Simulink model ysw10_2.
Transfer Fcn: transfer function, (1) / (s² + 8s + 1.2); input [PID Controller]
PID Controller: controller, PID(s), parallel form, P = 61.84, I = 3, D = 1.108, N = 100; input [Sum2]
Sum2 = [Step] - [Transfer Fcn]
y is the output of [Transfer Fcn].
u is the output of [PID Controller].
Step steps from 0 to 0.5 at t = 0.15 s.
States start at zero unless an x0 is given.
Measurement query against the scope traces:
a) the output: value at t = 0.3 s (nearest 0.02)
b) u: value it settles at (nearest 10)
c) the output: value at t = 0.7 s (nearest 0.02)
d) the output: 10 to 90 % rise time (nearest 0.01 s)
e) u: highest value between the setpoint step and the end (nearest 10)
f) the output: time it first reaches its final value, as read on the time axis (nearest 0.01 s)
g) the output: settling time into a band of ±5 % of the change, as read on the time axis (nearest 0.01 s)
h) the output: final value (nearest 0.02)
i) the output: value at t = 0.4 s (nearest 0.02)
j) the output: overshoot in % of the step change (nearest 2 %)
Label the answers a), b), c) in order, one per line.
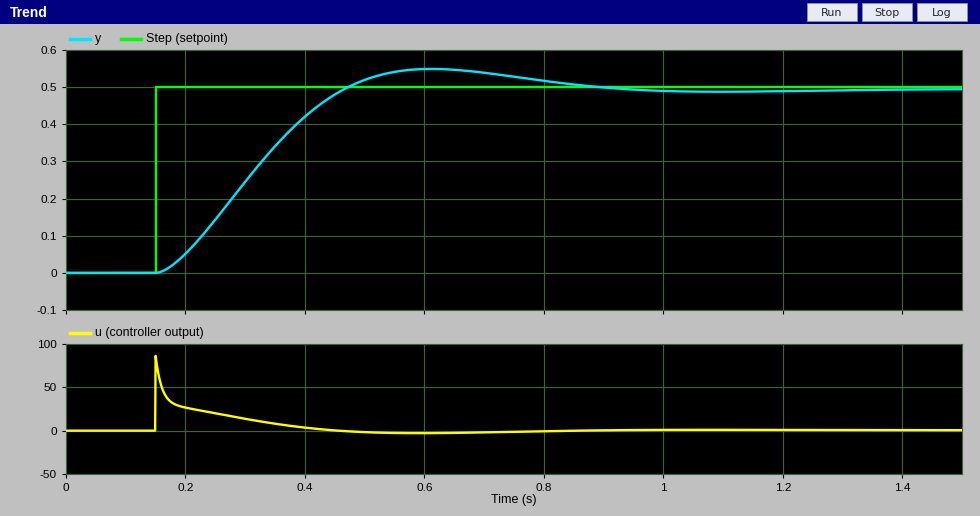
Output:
a) 0.24
b) 0
c) 0.54
d) 0.22 s
e) 90
f) 0.47 s
g) 0.79 s
h) 0.50
i) 0.42
j) 10 %
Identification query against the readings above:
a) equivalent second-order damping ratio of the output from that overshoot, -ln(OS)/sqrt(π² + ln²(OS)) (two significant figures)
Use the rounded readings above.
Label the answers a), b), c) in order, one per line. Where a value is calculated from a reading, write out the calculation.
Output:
a) ln(0.1) = -2.303; 2.303 / sqrt(9.870 + 5.302) = 0.59
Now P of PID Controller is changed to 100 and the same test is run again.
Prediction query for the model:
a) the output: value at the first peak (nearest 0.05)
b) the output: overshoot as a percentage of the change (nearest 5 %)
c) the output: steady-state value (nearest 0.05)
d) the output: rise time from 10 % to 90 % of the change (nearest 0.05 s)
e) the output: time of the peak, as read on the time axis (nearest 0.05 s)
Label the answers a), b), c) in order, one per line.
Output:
a) 0.60
b) 20 %
c) 0.50
d) 0.15 s
e) 0.50 s
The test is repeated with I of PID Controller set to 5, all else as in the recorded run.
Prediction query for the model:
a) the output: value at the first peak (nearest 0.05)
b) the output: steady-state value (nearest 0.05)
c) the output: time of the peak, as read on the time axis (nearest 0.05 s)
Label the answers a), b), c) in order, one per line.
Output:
a) 0.55
b) 0.50
c) 0.60 s
